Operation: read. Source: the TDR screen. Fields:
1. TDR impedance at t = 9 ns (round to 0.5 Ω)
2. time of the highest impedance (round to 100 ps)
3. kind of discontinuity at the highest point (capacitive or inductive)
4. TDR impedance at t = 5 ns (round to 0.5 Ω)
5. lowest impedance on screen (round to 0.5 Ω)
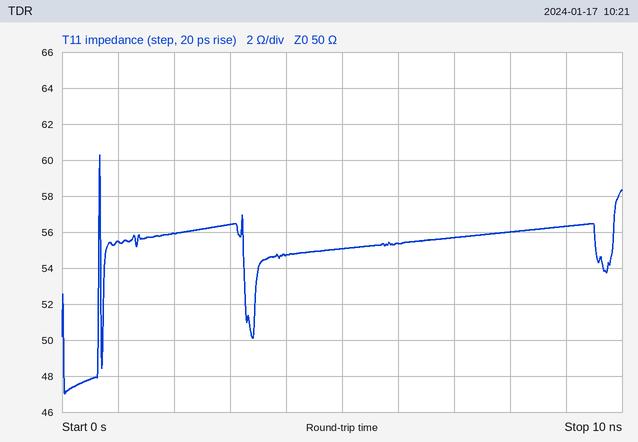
56.5 Ω
700 ps
inductive
55.0 Ω
47.0 Ω
